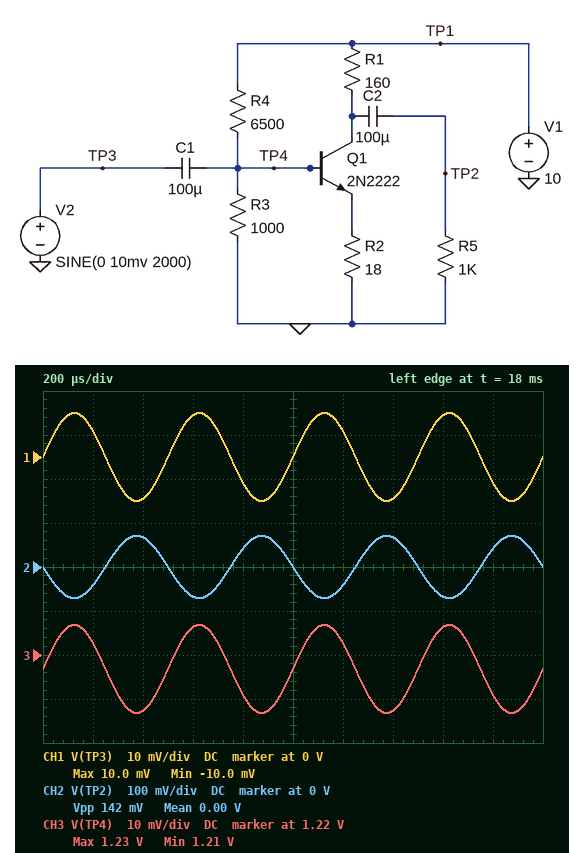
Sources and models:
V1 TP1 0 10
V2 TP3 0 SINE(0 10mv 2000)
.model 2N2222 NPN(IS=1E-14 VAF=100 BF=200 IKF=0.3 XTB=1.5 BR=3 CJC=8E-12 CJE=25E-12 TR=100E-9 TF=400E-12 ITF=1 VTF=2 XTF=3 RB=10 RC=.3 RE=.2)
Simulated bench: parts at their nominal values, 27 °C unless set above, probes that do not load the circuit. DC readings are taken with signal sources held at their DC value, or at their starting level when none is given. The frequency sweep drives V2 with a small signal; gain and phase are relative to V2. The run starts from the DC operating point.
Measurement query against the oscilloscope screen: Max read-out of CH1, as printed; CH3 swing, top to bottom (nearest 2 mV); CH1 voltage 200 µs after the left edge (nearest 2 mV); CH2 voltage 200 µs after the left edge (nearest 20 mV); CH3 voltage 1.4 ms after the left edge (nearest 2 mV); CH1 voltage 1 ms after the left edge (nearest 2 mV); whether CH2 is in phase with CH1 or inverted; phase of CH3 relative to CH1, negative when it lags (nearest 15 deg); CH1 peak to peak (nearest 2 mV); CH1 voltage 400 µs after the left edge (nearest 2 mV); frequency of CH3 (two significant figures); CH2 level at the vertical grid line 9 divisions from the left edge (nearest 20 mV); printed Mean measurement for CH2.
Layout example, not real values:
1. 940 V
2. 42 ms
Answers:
1. 10.0 mV
2. 20 mV
3. 6 mV
4. -40 mV
5. 1.208 V
6. 0 V
7. inverted
8. 0 deg
9. 20 mV
10. -10 mV
11. 2.0 kHz
12. 40 mV
13. 0.00 V
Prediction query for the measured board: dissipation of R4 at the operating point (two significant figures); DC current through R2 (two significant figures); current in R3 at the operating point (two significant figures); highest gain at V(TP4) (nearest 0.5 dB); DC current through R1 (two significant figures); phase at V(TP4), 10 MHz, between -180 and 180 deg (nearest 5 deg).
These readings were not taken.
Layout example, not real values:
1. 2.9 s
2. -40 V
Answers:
1. 12 mW
2. 26 mA
3. 1.2 mA
4. 0 dB
5. 26 mA
6. 0 deg
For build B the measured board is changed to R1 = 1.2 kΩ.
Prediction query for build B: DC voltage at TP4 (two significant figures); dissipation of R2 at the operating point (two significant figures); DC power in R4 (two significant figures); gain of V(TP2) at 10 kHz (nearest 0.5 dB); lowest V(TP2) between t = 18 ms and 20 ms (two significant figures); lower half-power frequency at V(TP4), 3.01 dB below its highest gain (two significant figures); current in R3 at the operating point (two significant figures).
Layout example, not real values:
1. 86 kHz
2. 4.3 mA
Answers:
1. 880 mV
2. 1.4 mW
3. 13 mW
4. -4.0 dB
5. -4.1 mV
6. 42 Hz
7. 880 µA
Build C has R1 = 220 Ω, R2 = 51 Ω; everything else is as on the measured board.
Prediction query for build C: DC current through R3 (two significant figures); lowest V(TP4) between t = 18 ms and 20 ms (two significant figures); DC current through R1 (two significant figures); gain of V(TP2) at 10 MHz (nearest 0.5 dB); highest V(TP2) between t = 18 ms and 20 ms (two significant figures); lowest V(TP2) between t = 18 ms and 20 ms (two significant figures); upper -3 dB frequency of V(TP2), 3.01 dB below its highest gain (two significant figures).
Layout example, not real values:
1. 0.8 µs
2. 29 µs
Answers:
1. 1.3 mA
2. 1.3 V
3. 11 mA
4. 10.5 dB
5. 33 mV
6. -33 mV
7. 170 MHz
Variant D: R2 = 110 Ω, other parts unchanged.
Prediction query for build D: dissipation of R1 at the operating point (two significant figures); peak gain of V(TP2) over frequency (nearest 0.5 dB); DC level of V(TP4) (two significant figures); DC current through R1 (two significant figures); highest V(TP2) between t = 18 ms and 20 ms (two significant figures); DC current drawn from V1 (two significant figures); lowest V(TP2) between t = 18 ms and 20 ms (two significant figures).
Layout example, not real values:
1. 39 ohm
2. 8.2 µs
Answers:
1. 4.9 mW
2. 1.5 dB
3. 1.3 V
4. 5.5 mA
5. 12 mV
6. 6.9 mA
7. -12 mV
